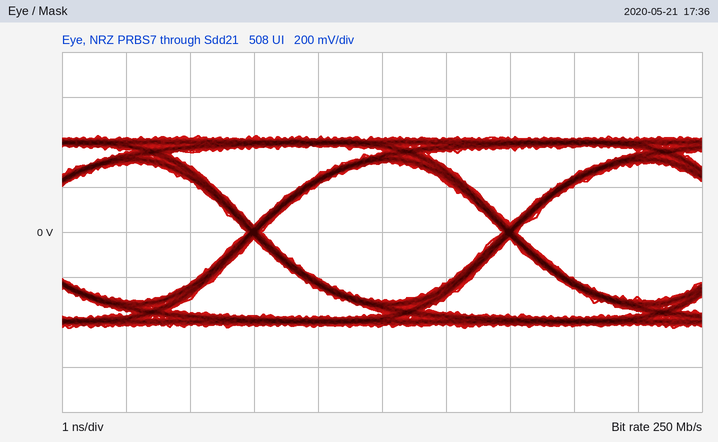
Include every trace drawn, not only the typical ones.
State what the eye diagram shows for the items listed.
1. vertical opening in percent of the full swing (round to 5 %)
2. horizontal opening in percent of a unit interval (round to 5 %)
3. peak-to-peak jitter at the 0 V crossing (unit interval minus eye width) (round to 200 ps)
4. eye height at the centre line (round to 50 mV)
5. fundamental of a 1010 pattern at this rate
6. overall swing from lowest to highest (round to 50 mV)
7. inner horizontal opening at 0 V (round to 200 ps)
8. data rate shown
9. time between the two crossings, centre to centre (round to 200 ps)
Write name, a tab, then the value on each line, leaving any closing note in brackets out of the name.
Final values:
vertical opening in percent of the full swing	70 %
horizontal opening in percent of a unit interval	95 %
peak-to-peak jitter at the 0 V crossing (unit interval minus eye width)	200 ps
eye height at the centre line	600 mV
fundamental of a 1010 pattern at this rate	125 MHz
overall swing from lowest to highest	850 mV
inner horizontal opening at 0 V	3.8 ns
data rate shown	250 Mb/s
time between the two crossings, centre to centre	4.0 ns
